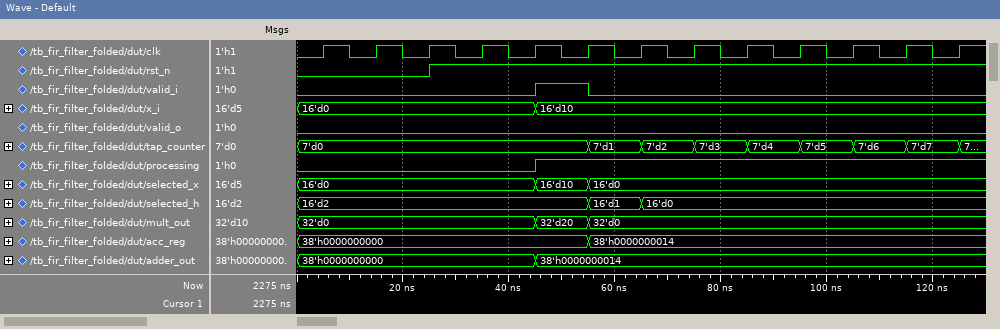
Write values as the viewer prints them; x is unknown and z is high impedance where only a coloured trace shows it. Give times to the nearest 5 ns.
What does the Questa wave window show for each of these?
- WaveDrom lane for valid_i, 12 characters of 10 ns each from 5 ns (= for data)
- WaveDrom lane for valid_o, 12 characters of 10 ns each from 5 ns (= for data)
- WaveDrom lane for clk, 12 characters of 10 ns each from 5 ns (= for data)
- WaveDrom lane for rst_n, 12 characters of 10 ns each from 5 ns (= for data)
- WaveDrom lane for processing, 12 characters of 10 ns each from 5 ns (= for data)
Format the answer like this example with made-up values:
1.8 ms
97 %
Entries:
{name: 'valid_i', wave: '0...10......'}
{name: 'valid_o', wave: '0...........'}
{name: 'clk', wave: 'p...........'}
{name: 'rst_n', wave: '0.1.........'}
{name: 'processing', wave: '0...1.......'}
